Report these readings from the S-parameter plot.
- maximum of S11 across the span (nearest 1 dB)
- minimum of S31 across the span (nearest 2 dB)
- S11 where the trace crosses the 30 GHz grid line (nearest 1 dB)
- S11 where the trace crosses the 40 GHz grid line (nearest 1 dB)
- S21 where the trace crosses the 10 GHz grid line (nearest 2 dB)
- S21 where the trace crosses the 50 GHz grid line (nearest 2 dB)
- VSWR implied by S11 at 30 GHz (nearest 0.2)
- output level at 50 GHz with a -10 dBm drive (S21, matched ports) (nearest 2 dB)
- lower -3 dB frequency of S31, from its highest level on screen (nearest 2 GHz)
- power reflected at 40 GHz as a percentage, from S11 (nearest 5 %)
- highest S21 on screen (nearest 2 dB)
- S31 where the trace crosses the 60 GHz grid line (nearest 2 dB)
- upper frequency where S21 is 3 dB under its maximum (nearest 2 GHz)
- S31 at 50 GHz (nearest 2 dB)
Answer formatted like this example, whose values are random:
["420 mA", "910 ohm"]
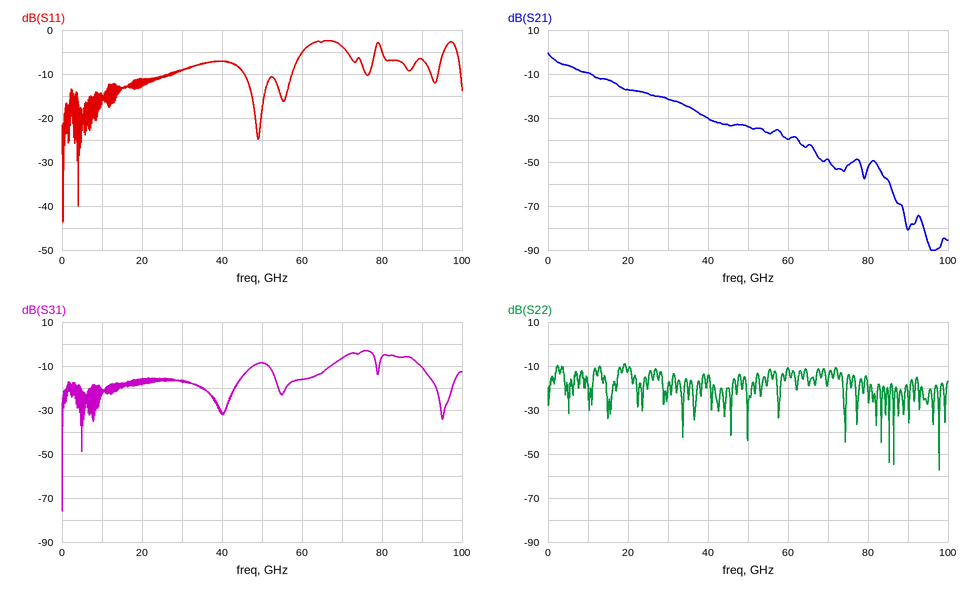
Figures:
["-2 dB", "-76 dB", "-9 dB", "-7 dB", "-10 dB", "-34 dB", "2.0", "-44 dBm", "70 GHz", "20 %", "0 dB", "-16 dB", "2 GHz", "-8 dB"]
